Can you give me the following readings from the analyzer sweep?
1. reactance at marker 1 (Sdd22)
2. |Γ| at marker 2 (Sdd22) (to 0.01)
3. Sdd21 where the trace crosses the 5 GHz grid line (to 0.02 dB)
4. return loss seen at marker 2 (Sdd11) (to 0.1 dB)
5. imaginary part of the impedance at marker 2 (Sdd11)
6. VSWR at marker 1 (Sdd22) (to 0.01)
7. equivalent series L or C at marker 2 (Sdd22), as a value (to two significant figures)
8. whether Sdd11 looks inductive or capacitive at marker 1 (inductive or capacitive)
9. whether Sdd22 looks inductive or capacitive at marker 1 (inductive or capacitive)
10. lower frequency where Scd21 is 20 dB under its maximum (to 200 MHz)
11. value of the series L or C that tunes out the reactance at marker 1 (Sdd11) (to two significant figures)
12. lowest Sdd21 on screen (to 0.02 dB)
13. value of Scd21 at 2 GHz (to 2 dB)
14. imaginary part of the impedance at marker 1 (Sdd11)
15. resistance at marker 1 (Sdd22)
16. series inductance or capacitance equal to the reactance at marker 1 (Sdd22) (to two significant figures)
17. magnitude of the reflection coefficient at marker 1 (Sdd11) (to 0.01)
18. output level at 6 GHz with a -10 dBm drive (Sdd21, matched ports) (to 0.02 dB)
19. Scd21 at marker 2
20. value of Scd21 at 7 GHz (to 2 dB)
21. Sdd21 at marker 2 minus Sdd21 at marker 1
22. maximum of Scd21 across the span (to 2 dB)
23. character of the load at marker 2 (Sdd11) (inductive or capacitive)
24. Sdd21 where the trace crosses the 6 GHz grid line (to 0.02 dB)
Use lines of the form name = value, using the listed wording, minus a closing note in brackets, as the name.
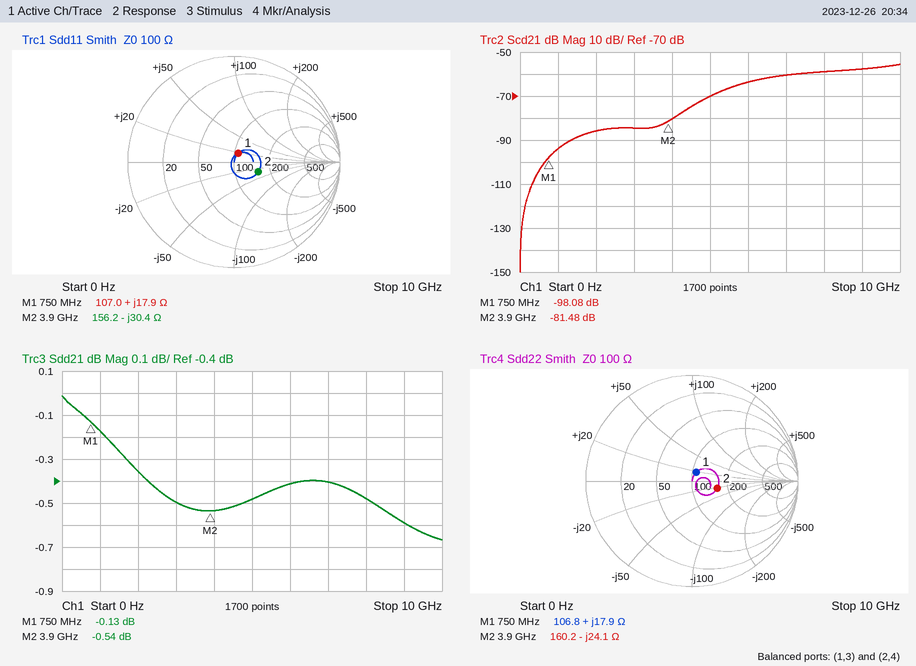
reactance at marker 1 = +17.9 Ω
|Γ| at marker 2 (Sdd22) = 0.25
Sdd21 where the trace crosses the 5 GHz grid line = -0.48 dB
return loss seen at marker 2 (Sdd11) = 12.1 dB
imaginary part of the impedance at marker 2 = -30.4 Ω
VSWR at marker 1 (Sdd22) = 1.20
equivalent series L or C at marker 2 (Sdd22), as a value = 1.7 pF
whether Sdd11 looks inductive or capacitive at marker 1 = inductive
whether Sdd22 looks inductive or capacitive at marker 1 = inductive
lower frequency where Scd21 is 20 dB under its maximum = 4.4 GHz
value of the series L or C that tunes out the reactance at marker 1 (Sdd11) = 12 pF
lowest Sdd21 on screen = -0.66 dB
value of Scd21 at 2 GHz = -86 dB
imaginary part of the impedance at marker 1 = +17.9 Ω
resistance at marker 1 = 106.8 Ω
series inductance or capacitance equal to the reactance at marker 1 (Sdd22) = 3.8 nH
magnitude of the reflection coefficient at marker 1 (Sdd11) = 0.09
output level at 6 GHz with a -10 dBm drive (Sdd21, matched ports) = -10.42 dBm
Scd21 at marker 2 = -81.48 dB
value of Scd21 at 7 GHz = -60 dB
Sdd21 at marker 2 minus Sdd21 at marker 1 = -0.41 dB
maximum of Scd21 across the span = -56 dB
character of the load at marker 2 (Sdd11) = capacitive
Sdd21 where the trace crosses the 6 GHz grid line = -0.42 dB
